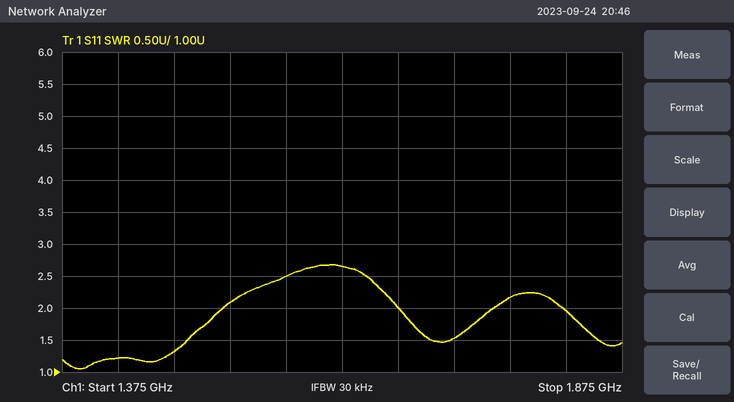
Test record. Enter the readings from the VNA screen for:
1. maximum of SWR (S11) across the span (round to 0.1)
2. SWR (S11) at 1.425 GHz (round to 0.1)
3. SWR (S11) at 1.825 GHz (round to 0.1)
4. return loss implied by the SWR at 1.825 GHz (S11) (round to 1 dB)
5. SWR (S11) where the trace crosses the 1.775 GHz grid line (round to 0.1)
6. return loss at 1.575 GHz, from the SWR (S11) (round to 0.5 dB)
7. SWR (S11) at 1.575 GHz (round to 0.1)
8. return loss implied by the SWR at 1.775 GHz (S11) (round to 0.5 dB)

2.7
1.2
2.0
10 dB
2.2
7.5 dB
2.5
8.5 dB
